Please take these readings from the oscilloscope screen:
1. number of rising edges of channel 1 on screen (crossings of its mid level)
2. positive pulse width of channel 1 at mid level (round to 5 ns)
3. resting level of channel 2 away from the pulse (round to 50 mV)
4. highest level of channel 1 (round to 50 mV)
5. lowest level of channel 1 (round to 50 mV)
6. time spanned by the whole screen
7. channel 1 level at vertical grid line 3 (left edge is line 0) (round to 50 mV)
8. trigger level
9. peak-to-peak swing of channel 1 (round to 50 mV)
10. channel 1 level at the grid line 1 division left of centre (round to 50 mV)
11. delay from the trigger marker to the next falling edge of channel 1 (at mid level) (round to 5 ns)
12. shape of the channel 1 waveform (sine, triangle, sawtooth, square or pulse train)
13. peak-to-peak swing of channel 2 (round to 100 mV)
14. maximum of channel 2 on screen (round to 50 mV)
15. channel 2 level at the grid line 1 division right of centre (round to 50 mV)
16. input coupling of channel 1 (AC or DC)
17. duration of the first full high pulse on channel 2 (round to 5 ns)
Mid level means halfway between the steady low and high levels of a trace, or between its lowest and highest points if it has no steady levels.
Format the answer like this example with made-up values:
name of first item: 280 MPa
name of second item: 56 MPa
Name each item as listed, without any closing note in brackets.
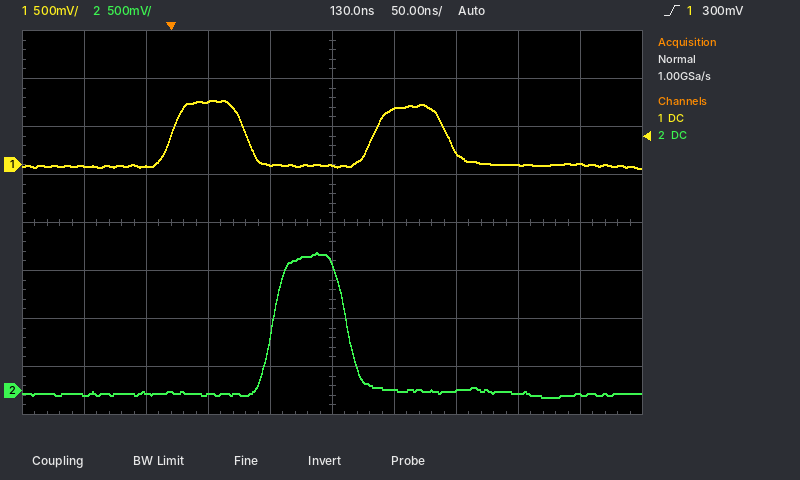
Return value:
number of rising edges of channel 1 on screen: 2
positive pulse width of channel 1 at mid level: 60 ns
resting level of channel 2 away from the pulse: -50 mV
highest level of channel 1: 650 mV
lowest level of channel 1: -50 mV
time spanned by the whole screen: 500 ns
channel 1 level at vertical grid line 3 (left edge is line 0): 650 mV
trigger level: 300 mV
peak-to-peak swing of channel 1: 700 mV
channel 1 level at the grid line 1 division left of centre: 0 mV
delay from the trigger marker to the next falling edge of channel 1 (at mid level): 60 ns
shape of the channel 1 waveform: pulse train
peak-to-peak swing of channel 2: 1.50 V
maximum of channel 2 on screen: 1.45 V
channel 2 level at the grid line 1 division right of centre: 0 mV
input coupling of channel 1: DC
duration of the first full high pulse on channel 2: 60 ns
